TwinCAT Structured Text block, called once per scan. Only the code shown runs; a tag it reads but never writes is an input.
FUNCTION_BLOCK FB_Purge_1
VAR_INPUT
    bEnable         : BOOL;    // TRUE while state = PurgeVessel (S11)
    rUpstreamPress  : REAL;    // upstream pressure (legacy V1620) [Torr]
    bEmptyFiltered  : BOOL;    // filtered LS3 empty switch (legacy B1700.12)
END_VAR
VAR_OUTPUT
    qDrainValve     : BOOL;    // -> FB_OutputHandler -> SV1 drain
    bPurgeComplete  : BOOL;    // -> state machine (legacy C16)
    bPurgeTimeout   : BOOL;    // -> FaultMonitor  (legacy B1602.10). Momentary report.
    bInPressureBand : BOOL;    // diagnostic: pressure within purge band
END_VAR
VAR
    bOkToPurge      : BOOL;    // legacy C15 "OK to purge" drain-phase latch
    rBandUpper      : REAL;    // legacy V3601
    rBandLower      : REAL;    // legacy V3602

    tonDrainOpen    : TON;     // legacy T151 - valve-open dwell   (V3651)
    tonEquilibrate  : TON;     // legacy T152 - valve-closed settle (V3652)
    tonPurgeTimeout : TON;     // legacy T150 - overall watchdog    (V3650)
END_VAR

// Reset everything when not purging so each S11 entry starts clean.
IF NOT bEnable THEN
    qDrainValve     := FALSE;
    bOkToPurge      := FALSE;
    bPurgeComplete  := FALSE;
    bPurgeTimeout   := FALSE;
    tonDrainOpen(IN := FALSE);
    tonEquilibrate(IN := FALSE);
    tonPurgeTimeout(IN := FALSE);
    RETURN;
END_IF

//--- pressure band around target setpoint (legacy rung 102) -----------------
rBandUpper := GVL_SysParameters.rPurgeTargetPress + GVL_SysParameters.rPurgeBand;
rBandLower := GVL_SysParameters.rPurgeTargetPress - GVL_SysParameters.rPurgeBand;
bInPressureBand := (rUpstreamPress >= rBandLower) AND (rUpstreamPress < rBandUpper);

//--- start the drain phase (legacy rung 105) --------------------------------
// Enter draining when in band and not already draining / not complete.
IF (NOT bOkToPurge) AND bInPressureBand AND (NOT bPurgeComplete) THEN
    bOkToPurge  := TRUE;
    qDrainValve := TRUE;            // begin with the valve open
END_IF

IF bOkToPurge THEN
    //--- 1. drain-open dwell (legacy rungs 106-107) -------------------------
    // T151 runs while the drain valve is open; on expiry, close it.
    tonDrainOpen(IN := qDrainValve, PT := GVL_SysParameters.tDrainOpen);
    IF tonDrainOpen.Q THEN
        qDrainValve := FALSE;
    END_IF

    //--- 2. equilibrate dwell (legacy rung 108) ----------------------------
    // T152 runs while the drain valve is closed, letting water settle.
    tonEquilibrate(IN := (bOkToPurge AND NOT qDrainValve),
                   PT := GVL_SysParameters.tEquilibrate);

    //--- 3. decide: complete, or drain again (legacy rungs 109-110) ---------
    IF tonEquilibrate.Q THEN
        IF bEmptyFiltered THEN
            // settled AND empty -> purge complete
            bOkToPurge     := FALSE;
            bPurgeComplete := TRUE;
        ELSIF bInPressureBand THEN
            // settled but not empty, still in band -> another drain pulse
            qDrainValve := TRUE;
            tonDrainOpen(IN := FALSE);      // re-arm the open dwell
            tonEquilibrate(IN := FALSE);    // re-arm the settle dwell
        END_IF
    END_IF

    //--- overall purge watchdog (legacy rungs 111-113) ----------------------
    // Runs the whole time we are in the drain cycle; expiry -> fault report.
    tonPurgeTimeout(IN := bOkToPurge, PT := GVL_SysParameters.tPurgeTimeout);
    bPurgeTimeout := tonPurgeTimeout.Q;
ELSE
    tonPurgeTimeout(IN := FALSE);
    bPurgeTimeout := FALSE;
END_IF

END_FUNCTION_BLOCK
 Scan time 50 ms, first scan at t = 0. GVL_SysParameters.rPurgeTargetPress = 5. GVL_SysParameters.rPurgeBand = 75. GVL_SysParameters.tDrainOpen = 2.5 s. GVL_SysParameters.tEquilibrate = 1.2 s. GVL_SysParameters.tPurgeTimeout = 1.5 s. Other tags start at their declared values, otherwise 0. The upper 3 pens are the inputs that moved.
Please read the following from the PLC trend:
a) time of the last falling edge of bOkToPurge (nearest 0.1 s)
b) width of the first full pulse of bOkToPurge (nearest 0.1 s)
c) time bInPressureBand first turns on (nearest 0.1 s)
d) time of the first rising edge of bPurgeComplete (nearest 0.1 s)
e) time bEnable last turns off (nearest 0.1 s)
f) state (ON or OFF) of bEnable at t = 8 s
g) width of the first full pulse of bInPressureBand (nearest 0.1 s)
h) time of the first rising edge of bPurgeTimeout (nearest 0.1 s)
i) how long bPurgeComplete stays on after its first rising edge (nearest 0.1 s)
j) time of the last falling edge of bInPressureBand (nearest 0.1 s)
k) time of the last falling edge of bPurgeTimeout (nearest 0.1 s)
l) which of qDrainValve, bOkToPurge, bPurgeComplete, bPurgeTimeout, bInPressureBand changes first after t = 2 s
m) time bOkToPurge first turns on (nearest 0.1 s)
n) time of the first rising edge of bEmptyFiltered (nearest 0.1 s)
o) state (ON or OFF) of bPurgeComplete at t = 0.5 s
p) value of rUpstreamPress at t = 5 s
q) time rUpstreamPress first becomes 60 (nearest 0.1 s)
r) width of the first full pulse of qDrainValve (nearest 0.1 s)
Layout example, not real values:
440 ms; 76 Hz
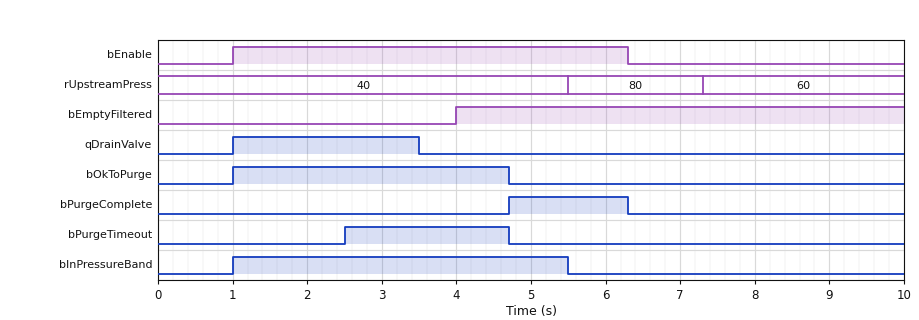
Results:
4.7 s; 3.7 s; 1.0 s; 4.7 s; 6.3 s; OFF; 4.5 s; 2.5 s; 1.6 s; 5.5 s; 4.7 s; bPurgeTimeout; 1.0 s; 4.0 s; OFF; 40; 7.3 s; 2.5 s
